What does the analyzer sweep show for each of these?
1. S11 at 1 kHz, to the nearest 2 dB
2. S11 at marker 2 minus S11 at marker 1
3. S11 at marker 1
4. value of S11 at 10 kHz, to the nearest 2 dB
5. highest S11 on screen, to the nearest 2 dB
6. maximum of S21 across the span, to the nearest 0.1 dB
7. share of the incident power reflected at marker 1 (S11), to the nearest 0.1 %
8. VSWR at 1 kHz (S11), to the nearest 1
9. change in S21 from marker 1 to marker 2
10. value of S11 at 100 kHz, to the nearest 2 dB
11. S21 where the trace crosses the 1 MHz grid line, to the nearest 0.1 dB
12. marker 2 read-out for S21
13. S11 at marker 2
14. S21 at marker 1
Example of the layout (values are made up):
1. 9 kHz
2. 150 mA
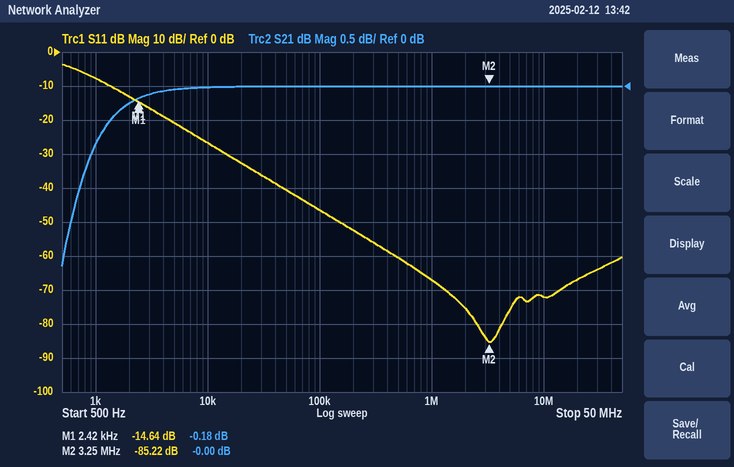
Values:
1. -8 dB
2. -70.58 dB
3. -14.64 dB
4. -26 dB
5. -4 dB
6. 0.0 dB
7. 3.4 %
8. 2
9. 0.18 dB
10. -46 dB
11. 0.0 dB
12. -0.00 dB
13. -85.22 dB
14. -0.18 dB
